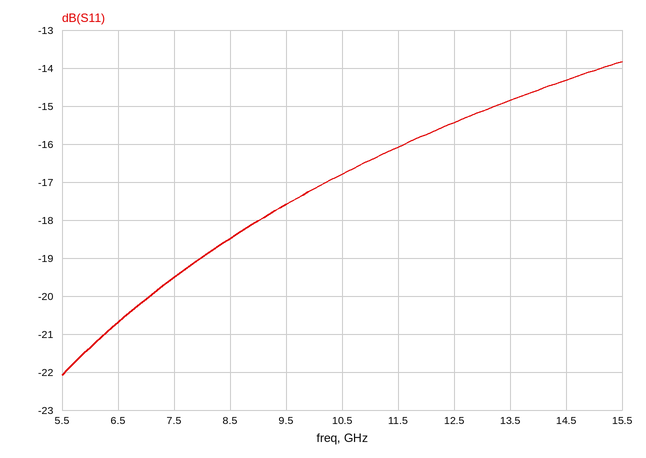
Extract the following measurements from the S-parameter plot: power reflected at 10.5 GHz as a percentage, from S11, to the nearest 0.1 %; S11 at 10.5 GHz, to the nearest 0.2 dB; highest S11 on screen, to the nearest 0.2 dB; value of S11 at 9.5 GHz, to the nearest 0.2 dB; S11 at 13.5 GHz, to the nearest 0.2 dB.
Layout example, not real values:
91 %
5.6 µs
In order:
2.1 %
-16.8 dB
-13.8 dB
-17.6 dB
-14.8 dB
